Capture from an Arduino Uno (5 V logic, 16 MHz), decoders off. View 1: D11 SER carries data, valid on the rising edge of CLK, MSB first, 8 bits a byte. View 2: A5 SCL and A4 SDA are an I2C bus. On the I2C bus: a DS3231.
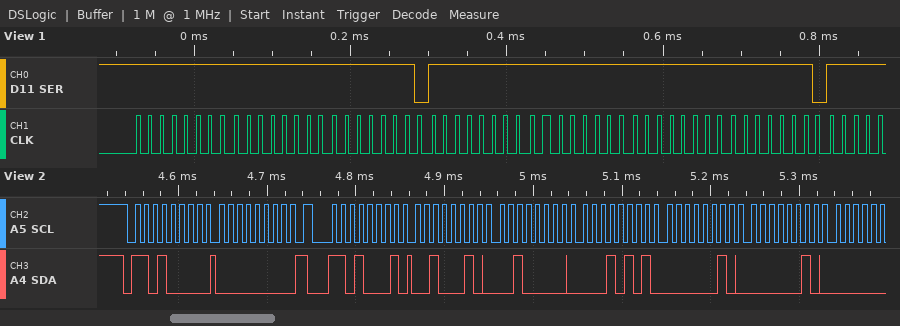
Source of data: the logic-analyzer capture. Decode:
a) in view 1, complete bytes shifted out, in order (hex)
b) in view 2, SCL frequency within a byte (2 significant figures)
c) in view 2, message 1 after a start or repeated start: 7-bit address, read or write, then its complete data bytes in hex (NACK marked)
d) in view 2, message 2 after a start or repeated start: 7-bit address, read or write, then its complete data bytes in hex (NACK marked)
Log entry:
FF FF FE FF FF FF FE
100 kHz
0x68 write: 00
0x68 read: 22 20 15 02 02
